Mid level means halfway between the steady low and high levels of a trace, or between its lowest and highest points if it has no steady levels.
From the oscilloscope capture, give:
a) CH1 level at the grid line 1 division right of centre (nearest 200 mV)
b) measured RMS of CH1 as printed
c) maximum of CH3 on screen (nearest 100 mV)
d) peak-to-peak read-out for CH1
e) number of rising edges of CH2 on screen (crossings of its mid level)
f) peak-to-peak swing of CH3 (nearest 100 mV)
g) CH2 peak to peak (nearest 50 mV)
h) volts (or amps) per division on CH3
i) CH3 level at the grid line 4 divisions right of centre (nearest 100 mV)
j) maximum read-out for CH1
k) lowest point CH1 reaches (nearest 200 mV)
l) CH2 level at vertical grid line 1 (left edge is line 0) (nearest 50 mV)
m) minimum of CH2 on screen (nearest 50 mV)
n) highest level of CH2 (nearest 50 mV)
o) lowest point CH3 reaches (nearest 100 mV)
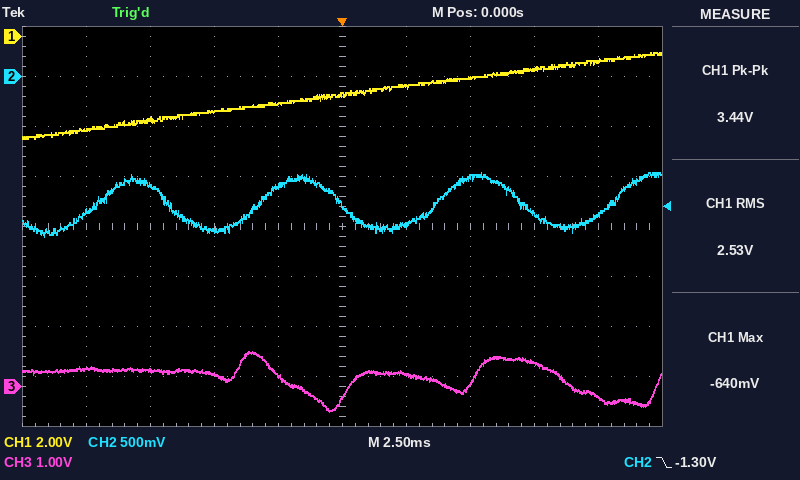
-2.0 V
2.53 V
700 mV
3.44 V
4
1.2 V
650 mV
1 V
-200 mV
-640 mV
-4.0 V
-1.35 V
-1.60 V
-950 mV
-500 mV
